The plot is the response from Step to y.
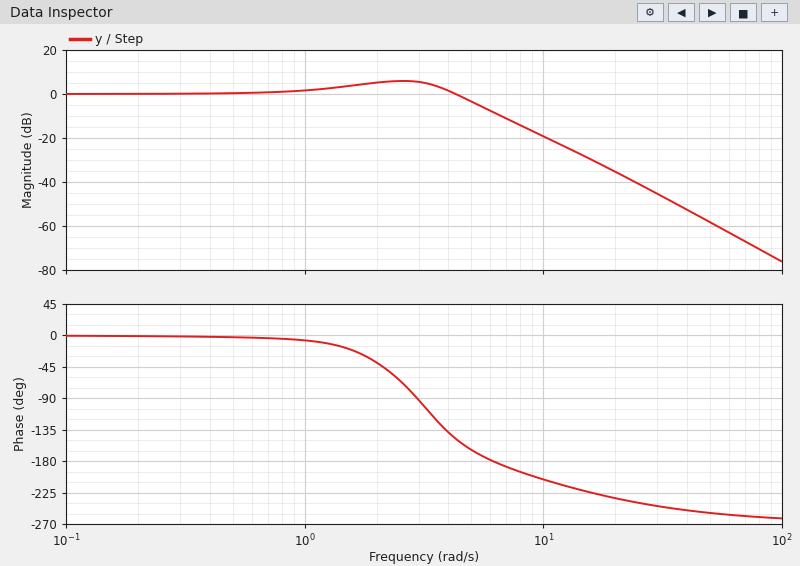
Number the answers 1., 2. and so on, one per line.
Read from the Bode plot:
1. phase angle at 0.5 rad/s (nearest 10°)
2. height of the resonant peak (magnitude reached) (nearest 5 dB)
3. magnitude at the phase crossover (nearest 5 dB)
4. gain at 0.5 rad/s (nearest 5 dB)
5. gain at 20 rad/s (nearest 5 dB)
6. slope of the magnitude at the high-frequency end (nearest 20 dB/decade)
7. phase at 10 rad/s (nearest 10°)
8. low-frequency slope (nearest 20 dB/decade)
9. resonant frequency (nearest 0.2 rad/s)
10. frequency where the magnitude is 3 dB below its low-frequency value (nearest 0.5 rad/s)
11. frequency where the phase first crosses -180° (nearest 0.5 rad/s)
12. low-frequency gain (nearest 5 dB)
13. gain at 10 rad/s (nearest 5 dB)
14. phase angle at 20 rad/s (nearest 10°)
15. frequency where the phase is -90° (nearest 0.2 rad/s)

1. 0°
2. 5 dB
3. -10 dB
4. 0 dB
5. -35 dB
6. -60 dB/decade
7. -210°
8. 0 dB/decade
9. 2.6 rad/s
10. 5.0 rad/s
11. 6.0 rad/s
12. 0 dB
13. -20 dB
14. -230°
15. 3.0 rad/s
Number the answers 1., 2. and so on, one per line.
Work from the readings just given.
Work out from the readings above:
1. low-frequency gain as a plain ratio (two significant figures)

1. 1.0
